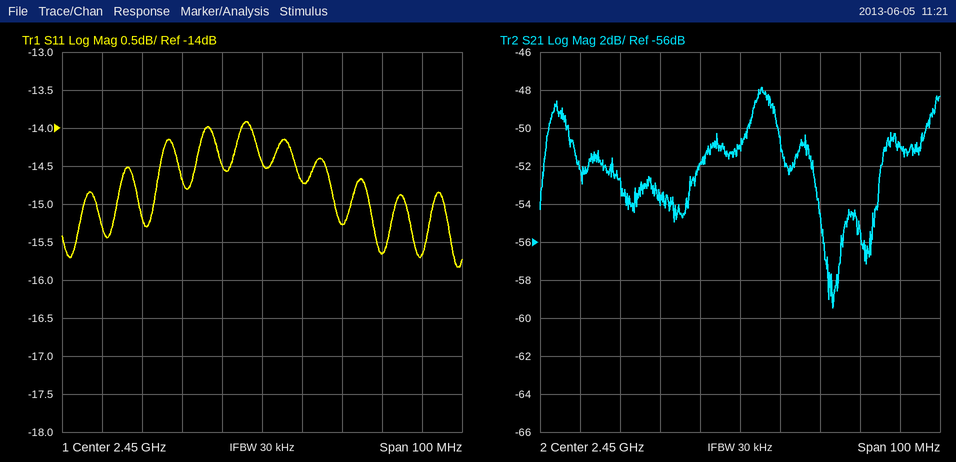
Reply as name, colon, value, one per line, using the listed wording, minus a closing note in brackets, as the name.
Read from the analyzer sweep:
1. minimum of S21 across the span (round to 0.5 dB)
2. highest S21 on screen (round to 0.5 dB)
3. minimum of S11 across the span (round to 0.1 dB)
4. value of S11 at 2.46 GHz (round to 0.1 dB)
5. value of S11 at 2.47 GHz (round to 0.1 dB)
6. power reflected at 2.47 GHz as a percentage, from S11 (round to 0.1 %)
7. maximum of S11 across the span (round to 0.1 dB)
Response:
minimum of S21 across the span: -59.5 dB
highest S21 on screen: -48.0 dB
minimum of S11 across the span: -15.8 dB
value of S11 at 2.46 GHz: -14.7 dB
value of S11 at 2.47 GHz: -15.3 dB
power reflected at 2.47 GHz as a percentage, from S11: 3.0 %
maximum of S11 across the span: -13.9 dB
